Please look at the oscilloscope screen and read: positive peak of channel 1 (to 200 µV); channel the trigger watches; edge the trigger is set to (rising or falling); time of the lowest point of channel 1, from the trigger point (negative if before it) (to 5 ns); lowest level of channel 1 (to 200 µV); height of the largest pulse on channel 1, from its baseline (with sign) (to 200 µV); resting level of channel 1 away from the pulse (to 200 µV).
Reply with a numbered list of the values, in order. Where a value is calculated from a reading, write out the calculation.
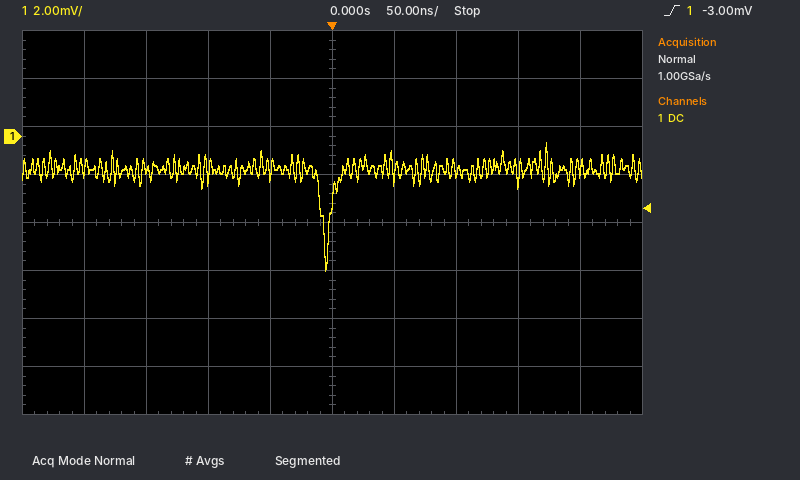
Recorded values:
1. -200 µV
2. channel 1
3. rising
4. -5 ns
5. -5.6 mV
6. -5.6 mV − (-1.4 mV) = -4.2 mV
7. -1.4 mV
